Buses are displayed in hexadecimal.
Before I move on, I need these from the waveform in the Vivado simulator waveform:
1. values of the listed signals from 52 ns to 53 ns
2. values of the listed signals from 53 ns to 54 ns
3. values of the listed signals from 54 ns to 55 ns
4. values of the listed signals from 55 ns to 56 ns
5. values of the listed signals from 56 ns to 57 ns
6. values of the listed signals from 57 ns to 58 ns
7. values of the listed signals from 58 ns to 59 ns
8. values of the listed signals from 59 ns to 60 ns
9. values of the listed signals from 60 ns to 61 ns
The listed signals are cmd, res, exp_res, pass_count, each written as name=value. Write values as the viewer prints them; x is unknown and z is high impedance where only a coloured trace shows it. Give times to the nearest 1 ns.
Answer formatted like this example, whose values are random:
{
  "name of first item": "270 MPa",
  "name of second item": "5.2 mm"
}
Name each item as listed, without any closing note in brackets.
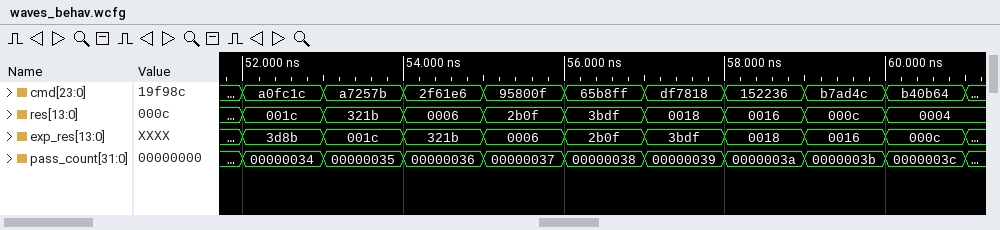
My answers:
{
  "values of the listed signals from 52 ns to 53 ns": "cmd=a0fc1c, res=001c, exp_res=3d8b, pass_count=00000034",
  "values of the listed signals from 53 ns to 54 ns": "cmd=a7257b, res=321b, exp_res=001c, pass_count=00000035",
  "values of the listed signals from 54 ns to 55 ns": "cmd=2f61e6, res=0006, exp_res=321b, pass_count=00000036",
  "values of the listed signals from 55 ns to 56 ns": "cmd=95800f, res=2b0f, exp_res=0006, pass_count=00000037",
  "values of the listed signals from 56 ns to 57 ns": "cmd=65b8ff, res=3bdf, exp_res=2b0f, pass_count=00000038",
  "values of the listed signals from 57 ns to 58 ns": "cmd=df7818, res=0018, exp_res=3bdf, pass_count=00000039",
  "values of the listed signals from 58 ns to 59 ns": "cmd=152236, res=0016, exp_res=0018, pass_count=0000003a",
  "values of the listed signals from 59 ns to 60 ns": "cmd=b7ad4c, res=000c, exp_res=0016, pass_count=0000003b",
  "values of the listed signals from 60 ns to 61 ns": "cmd=b40b64, res=0004, exp_res=000c, pass_count=0000003c"
}
